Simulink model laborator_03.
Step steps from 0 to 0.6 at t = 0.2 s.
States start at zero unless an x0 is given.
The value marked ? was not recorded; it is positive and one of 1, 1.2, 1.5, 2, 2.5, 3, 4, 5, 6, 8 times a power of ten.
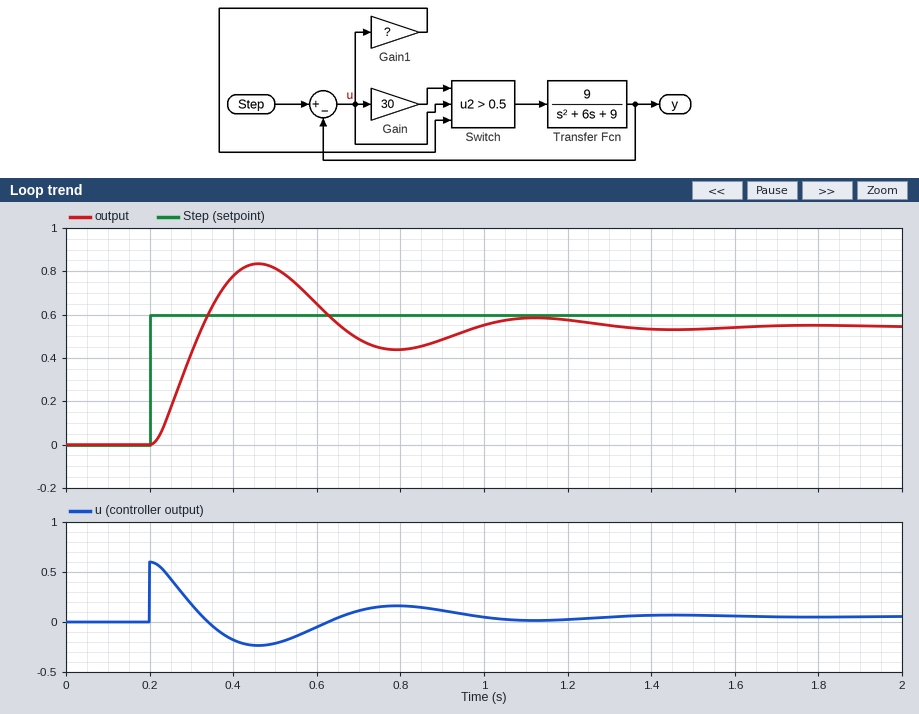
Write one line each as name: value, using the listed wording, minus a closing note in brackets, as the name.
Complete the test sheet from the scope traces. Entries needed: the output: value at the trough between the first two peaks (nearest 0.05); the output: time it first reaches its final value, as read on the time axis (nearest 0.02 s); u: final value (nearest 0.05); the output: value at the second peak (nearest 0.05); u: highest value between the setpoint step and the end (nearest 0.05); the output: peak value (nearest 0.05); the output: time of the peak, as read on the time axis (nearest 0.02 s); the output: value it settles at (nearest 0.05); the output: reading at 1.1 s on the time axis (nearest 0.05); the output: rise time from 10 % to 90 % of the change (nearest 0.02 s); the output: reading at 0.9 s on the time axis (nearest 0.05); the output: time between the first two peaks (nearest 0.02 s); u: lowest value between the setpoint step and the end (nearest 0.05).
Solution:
the output: value at the trough between the first two peaks: 0.45
the output: time it first reaches its final value, as read on the time axis: 0.32 s
u: final value: 0.05
the output: value at the second peak: 0.60
u: highest value between the setpoint step and the end: 0.60
the output: peak value: 0.85
the output: time of the peak, as read on the time axis: 0.46 s
the output: value it settles at: 0.55
the output: reading at 1.1 s on the time axis: 0.60
the output: rise time from 10 % to 90 % of the change: 0.08 s
the output: reading at 0.9 s on the time axis: 0.50
the output: time between the first two peaks: 0.66 s
u: lowest value between the setpoint step and the end: -0.25
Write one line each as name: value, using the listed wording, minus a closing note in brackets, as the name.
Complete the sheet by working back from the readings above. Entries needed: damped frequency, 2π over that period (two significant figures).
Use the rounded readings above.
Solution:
damped frequency, 2π over that period: 9.5 rad/s
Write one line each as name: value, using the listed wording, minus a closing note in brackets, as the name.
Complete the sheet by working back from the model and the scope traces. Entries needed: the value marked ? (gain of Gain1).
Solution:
the value marked ?: 10
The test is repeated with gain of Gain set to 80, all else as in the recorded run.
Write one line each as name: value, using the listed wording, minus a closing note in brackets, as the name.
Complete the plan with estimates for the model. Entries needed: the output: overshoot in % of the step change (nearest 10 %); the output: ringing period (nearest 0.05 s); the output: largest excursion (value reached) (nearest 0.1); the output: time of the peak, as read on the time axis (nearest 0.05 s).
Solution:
the output: overshoot in % of the step change: 90 %
the output: ringing period: 0.65 s
the output: largest excursion (value reached): 1.0
the output: time of the peak, as read on the time axis: 0.40 s
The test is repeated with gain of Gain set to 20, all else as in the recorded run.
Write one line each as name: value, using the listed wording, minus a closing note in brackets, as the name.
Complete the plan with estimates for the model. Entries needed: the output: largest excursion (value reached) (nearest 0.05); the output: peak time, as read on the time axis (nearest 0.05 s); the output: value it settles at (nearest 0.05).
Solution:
the output: largest excursion (value reached): 0.80
the output: peak time, as read on the time axis: 0.50 s
the output: value it settles at: 0.55
